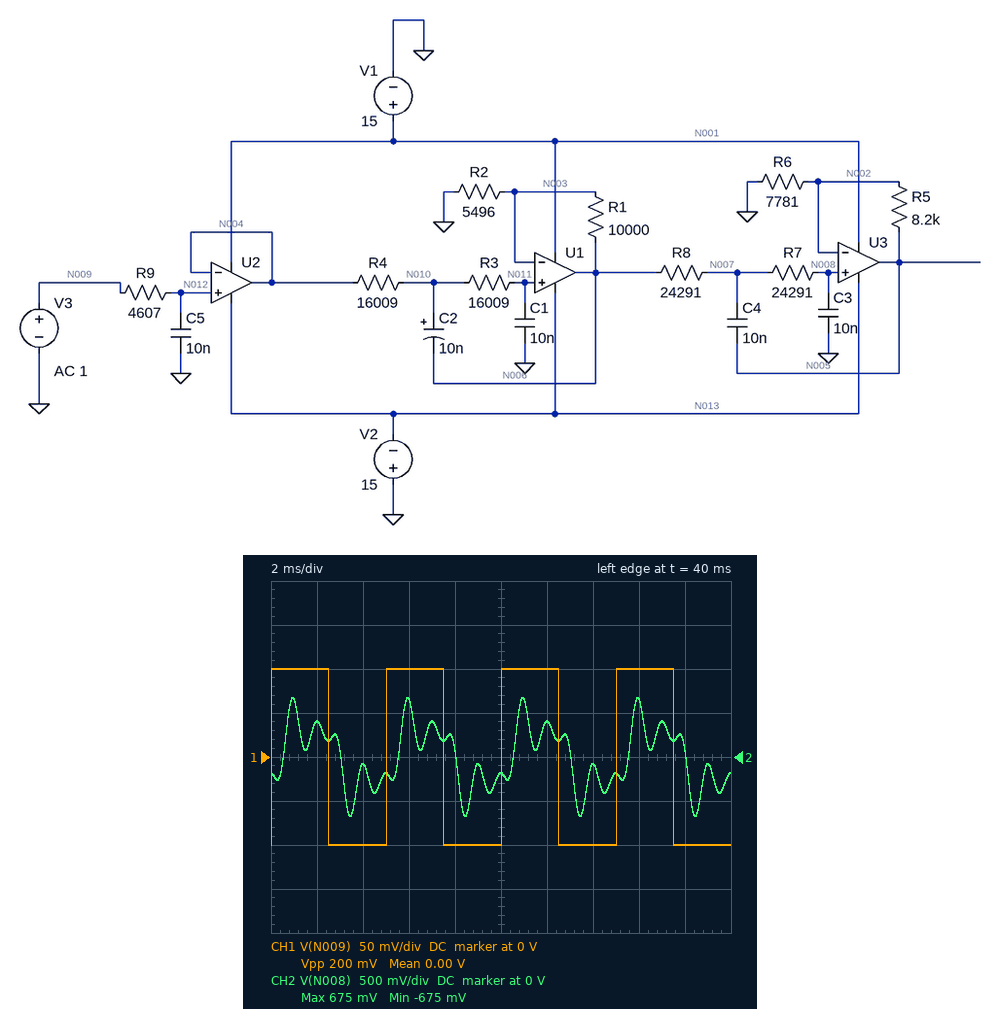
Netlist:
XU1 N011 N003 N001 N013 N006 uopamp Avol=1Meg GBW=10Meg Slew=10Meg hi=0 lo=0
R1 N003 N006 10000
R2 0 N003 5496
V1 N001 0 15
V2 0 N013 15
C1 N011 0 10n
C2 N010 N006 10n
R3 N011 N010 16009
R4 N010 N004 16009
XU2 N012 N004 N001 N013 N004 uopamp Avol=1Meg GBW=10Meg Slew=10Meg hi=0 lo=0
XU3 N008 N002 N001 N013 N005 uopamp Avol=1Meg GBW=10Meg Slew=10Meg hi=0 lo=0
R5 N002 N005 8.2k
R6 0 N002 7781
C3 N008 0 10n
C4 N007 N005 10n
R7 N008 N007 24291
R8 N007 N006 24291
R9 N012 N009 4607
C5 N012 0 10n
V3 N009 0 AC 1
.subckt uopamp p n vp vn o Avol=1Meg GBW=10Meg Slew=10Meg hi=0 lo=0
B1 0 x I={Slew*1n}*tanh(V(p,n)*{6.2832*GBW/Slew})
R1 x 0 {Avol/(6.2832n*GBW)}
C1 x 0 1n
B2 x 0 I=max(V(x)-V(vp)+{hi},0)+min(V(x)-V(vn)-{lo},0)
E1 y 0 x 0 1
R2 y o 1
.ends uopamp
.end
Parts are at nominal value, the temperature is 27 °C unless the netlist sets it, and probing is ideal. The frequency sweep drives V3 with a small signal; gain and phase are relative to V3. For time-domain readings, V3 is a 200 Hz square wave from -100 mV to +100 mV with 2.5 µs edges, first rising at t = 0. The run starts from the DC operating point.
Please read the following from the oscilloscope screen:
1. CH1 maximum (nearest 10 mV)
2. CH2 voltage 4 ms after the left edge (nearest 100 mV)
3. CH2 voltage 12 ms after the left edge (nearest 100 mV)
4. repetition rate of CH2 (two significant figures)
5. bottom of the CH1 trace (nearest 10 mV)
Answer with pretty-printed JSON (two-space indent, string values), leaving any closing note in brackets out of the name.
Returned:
{
  "CH1 maximum": "100 mV",
  "CH2 voltage 4 ms after the left edge": "-100 mV",
  "CH2 voltage 12 ms after the left edge": "400 mV",
  "repetition rate of CH2": "200 Hz",
  "bottom of the CH1 trace": "-100 mV"
}
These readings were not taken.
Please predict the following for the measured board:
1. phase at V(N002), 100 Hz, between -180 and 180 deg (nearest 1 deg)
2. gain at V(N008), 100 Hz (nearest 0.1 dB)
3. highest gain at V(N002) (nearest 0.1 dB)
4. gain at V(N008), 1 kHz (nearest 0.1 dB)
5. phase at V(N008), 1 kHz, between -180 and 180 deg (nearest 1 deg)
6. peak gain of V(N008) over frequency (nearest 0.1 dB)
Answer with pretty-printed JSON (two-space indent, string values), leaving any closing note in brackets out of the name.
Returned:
{
  "phase at V(N002), 100 Hz, between -180 and 180 deg": "-11 deg",
  "gain at V(N008), 100 Hz": "9.2 dB",
  "highest gain at V(N002)": "18.2 dB",
  "gain at V(N008), 1 kHz": "17.6 dB",
  "phase at V(N008), 1 kHz, between -180 and 180 deg": "117 deg",
  "peak gain of V(N008) over frequency": "18.2 dB"
}
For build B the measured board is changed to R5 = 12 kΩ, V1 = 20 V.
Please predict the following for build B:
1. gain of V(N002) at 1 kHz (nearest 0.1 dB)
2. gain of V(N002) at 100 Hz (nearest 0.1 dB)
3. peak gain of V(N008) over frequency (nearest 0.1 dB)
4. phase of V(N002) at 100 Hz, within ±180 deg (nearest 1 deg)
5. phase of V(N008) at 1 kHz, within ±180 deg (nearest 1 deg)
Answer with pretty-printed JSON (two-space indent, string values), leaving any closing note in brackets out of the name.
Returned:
{
  "gain of V(N002) at 1 kHz": "19.9 dB",
  "gain of V(N002) at 100 Hz": "9.3 dB",
  "peak gain of V(N008) over frequency": "20.8 dB",
  "phase of V(N002) at 100 Hz, within ±180 deg": "-7 deg",
  "phase of V(N008) at 1 kHz, within ±180 deg": "98 deg"
}
